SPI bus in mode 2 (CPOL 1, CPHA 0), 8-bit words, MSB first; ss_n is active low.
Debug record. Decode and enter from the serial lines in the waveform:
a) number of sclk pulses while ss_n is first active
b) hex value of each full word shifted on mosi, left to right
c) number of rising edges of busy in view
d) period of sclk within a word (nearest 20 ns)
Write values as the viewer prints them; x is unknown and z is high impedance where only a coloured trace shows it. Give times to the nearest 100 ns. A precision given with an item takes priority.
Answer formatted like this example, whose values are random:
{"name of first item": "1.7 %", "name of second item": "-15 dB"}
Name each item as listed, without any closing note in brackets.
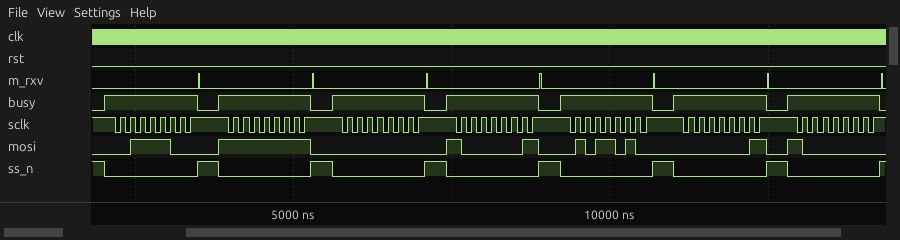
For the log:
{"number of sclk pulses while ss_n is first active": "8", "hex value of each full word shifted on mosi, left to right": "3C, FF, 00, 81, 5A, 01, 80", "number of rising edges of busy in view": "7", "period of sclk within a word": "160 ns"}
